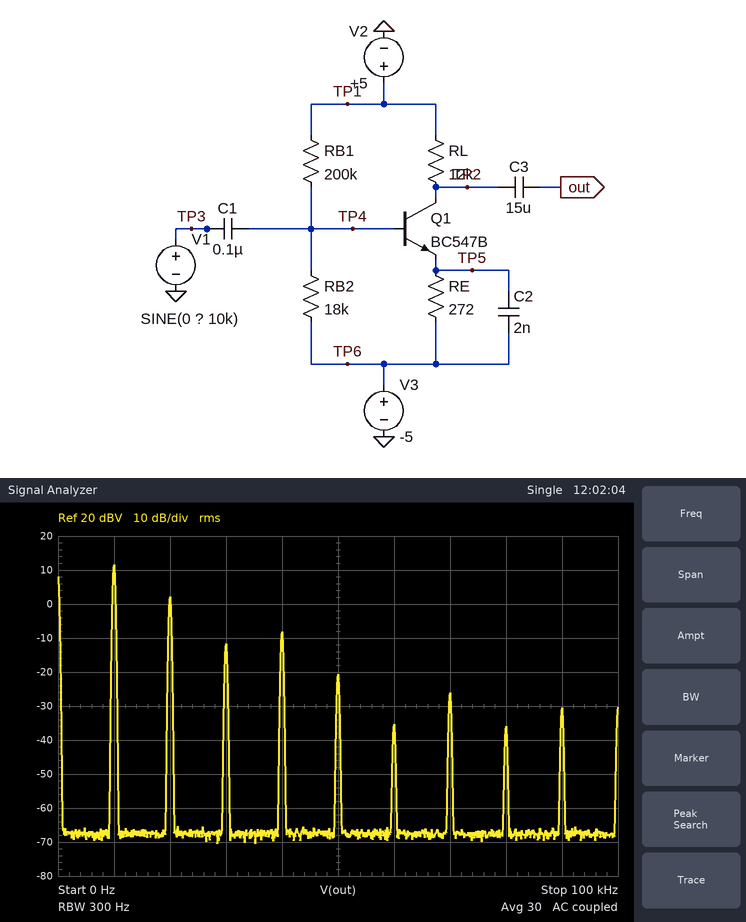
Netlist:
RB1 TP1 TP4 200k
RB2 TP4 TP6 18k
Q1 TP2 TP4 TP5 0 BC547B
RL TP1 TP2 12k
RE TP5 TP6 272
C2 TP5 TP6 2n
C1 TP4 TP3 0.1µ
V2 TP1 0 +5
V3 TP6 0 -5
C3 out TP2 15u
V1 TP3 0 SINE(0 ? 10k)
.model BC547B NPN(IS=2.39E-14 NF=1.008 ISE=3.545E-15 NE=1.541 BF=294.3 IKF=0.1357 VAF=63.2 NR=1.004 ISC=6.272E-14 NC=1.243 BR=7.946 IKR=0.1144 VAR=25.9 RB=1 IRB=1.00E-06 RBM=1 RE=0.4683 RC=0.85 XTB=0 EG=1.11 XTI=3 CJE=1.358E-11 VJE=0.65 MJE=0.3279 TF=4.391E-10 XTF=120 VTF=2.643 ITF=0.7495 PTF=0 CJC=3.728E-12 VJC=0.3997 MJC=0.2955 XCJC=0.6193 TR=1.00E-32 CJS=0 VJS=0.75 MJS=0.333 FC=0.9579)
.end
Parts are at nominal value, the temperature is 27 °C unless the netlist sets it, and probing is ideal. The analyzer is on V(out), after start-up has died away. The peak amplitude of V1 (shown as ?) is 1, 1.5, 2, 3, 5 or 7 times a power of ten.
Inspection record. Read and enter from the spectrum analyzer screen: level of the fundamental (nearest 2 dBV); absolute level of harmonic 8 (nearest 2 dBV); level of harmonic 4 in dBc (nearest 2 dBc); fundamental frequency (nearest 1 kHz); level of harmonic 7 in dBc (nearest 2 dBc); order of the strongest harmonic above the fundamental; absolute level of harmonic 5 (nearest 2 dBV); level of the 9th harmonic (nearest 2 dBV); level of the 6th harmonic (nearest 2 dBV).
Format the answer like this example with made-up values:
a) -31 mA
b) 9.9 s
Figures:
a) 12 dBV
b) -36 dBV
c) -20 dBc
d) 10 kHz
e) -38 dBc
f) 2
g) -20 dBV
h) -30 dBV
i) -36 dBV
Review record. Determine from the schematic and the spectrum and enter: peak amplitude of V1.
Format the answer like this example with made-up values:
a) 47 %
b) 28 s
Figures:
a) 300 mV
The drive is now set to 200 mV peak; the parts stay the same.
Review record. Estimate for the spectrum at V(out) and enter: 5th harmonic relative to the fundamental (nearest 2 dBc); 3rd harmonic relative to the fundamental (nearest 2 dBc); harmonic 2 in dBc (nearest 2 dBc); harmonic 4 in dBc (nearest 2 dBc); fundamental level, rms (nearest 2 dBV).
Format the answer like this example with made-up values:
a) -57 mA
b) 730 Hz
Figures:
a) -36 dBc
b) -22 dBc
c) -18 dBc
d) -32 dBc
e) 12 dBV
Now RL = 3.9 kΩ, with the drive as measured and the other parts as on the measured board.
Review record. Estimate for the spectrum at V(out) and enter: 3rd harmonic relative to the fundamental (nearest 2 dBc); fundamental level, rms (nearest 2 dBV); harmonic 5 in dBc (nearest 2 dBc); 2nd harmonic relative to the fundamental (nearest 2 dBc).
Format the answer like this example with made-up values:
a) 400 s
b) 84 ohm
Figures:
a) -26 dBc
b) 8 dBV
c) -56 dBc
d) -18 dBc
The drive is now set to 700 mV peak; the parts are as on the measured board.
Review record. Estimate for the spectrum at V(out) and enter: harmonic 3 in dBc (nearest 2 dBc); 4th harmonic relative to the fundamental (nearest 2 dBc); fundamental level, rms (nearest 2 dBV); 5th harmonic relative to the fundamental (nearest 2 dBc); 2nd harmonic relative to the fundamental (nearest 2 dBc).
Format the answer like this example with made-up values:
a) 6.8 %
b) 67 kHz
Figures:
a) -14 dBc
b) -22 dBc
c) 10 dBV
d) -16 dBc
e) -4 dBc
